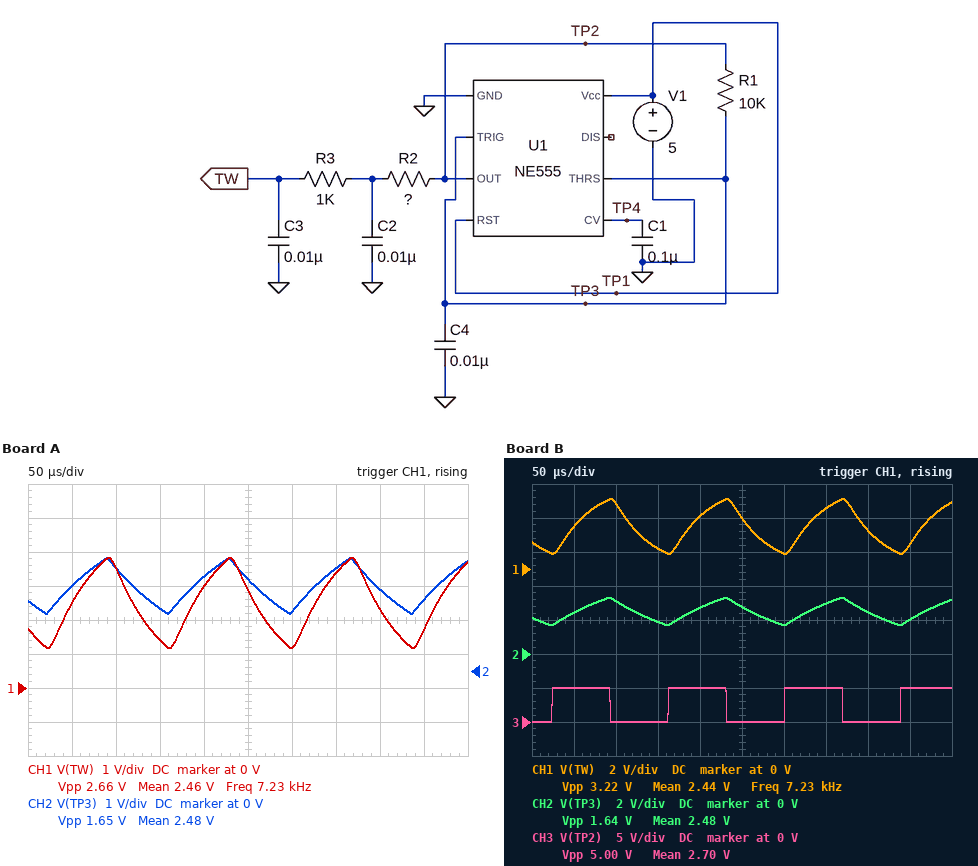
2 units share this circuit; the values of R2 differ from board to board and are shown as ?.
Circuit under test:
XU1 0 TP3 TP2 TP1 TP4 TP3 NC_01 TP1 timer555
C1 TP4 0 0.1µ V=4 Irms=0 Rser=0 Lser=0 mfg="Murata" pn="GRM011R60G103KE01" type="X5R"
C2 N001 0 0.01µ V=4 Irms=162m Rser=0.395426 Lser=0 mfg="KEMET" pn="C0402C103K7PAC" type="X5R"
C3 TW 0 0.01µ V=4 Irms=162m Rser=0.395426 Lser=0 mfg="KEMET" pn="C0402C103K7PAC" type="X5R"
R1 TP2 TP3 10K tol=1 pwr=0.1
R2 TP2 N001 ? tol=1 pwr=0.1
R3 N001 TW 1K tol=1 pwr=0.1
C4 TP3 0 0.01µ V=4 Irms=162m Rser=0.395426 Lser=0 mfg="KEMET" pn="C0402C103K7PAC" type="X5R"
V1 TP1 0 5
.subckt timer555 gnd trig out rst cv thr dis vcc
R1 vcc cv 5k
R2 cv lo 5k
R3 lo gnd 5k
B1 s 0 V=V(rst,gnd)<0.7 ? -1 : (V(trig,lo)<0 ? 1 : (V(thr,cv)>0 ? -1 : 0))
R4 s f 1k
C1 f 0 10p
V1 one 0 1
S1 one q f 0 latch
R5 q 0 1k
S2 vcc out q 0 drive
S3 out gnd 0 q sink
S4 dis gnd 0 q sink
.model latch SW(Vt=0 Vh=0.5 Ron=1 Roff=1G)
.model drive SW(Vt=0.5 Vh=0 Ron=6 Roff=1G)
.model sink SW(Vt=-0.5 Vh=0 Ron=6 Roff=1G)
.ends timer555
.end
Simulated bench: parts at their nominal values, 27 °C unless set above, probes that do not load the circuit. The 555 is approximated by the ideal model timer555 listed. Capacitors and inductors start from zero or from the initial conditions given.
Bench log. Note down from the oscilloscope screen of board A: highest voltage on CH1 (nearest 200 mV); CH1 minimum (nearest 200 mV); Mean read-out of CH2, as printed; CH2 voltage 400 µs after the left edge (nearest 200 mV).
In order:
3.8 V
1.2 V
2.48 V
2.4 V
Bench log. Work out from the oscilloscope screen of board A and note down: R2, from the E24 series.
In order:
2.4 kΩ
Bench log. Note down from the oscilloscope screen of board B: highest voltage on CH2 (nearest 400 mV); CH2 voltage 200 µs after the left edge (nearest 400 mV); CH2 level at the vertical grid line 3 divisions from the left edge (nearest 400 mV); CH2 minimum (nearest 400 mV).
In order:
3.2 V
2.8 V
2.0 V
1.6 V
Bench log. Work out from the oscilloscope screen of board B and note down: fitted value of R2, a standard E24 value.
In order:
1.8 kΩ
